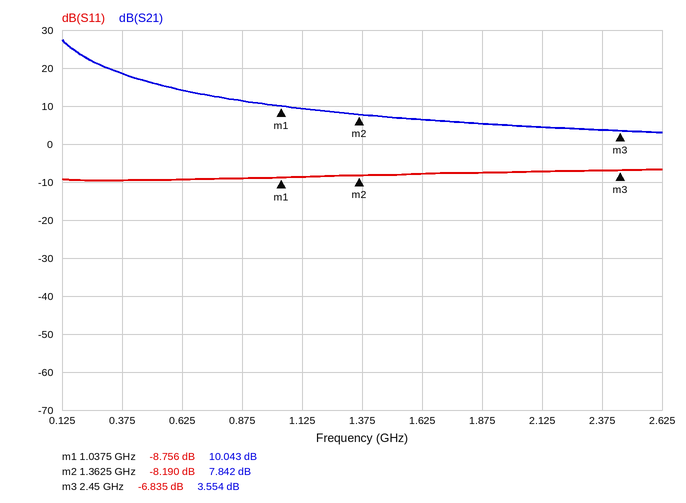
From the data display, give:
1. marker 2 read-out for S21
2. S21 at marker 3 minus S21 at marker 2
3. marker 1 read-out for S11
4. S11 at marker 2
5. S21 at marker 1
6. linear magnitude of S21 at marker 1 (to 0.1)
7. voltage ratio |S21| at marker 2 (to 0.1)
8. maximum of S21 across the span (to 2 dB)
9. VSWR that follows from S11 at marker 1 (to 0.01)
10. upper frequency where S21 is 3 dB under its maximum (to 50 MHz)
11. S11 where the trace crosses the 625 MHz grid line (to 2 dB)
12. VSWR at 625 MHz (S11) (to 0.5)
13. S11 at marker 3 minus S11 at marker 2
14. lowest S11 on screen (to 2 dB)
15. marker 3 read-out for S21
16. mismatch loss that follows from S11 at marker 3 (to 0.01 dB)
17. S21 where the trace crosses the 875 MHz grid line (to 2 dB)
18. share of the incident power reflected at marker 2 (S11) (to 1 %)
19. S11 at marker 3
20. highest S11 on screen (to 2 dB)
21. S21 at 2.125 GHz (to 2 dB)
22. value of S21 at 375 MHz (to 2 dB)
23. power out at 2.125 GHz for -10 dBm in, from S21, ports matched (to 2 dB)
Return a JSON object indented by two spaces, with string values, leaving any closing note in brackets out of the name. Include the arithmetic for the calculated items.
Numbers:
{
  "marker 2 read-out for S21": "7.842 dB",
  "S21 at marker 3 minus S21 at marker 2": "3.554 − (7.842) = -4.288 dB",
  "marker 1 read-out for S11": "-8.756 dB",
  "S11 at marker 2": "-8.190 dB",
  "S21 at marker 1": "10.043 dB",
  "linear magnitude of S21 at marker 1": "10^(10.043/20) ≈ 3.2",
  "voltage ratio |S21| at marker 2": "10^(7.842/20) ≈ 2.5",
  "maximum of S21 across the span": "28 dB",
  "VSWR that follows from S11 at marker 1": "(1 + 0.3649)/(1 − 0.3649) ≈ 2.15",
  "upper frequency where S21 is 3 dB under its maximum": "200 MHz",
  "S11 where the trace crosses the 625 MHz grid line": "-10 dB",
  "VSWR at 625 MHz (S11)": "|Γ| = 10^(-10/20) = 0.3162; VSWR = (1 + 0.3162)/(1 − 0.3162) ≈ 1.92, so 2.0 to the nearest 0.5",
  "S11 at marker 3 minus S11 at marker 2": "-6.835 − (-8.19) = 1.355 dB",
  "lowest S11 on screen": "-10 dB",
  "marker 3 read-out for S21": "3.554 dB",
  "mismatch loss that follows from S11 at marker 3": "−10 log10(1 − 10^(-6.835/10)) ≈ 1.01 dB",
  "S21 where the trace crosses the 875 MHz grid line": "12 dB",
  "share of the incident power reflected at marker 2 (S11)": "10^(-8.19/10) ≈ 15 %",
  "S11 at marker 3": "-6.835 dB",
  "highest S11 on screen": "-6 dB",
  "S21 at 2.125 GHz": "4 dB",
  "value of S21 at 375 MHz": "18 dB",
  "power out at 2.125 GHz for -10 dBm in, from S21, ports matched": "-10 dBm + (4 dB) = -6 dBm"
}
